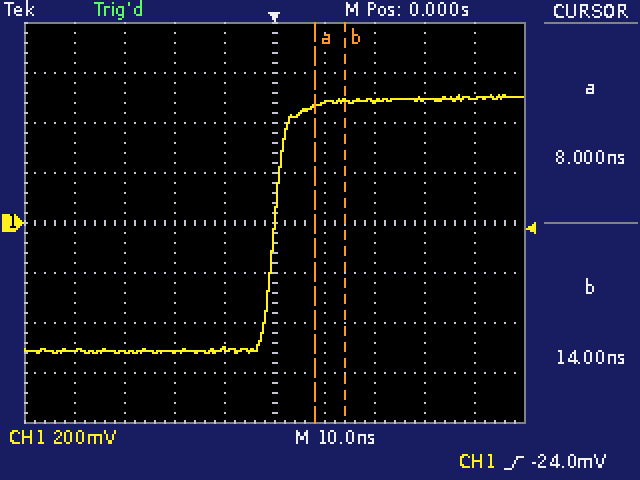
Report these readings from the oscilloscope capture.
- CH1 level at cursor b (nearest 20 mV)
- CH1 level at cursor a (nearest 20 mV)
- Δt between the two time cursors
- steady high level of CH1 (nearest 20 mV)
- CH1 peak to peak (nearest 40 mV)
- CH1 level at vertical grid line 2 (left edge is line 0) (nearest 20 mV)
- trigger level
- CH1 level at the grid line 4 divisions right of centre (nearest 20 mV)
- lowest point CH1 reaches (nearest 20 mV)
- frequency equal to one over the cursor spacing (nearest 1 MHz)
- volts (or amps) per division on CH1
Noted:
480 mV
460 mV
6 ns
500 mV
1.04 V
-520 mV
-24.0 mV
500 mV
-520 mV
167 MHz
200 mV
